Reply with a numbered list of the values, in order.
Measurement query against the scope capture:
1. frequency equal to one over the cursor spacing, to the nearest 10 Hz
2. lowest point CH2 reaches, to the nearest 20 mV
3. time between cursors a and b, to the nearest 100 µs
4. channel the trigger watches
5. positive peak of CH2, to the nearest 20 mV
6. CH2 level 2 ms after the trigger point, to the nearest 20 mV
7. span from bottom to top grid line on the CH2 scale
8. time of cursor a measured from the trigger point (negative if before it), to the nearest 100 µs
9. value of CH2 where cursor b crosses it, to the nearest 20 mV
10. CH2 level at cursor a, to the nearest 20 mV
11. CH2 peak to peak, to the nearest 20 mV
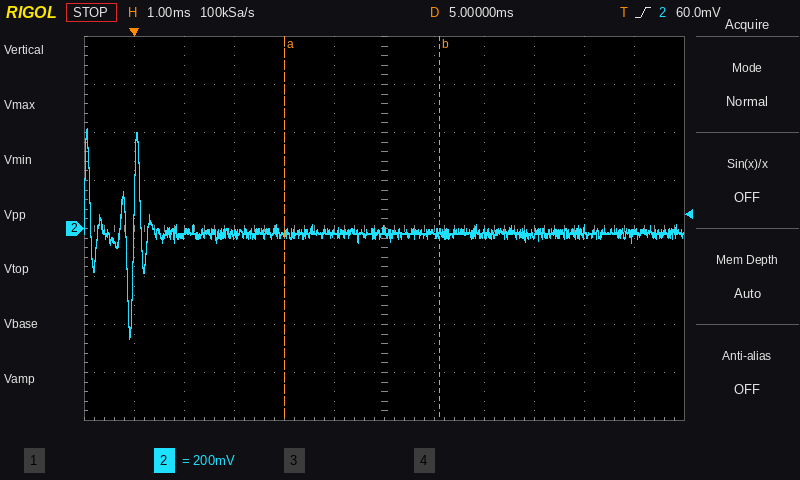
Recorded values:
1. 320 Hz
2. -460 mV
3. 3.1 ms
4. CH2
5. 420 mV
6. -20 mV
7. 1.6 V
8. +3.0 ms
9. -20 mV
10. -20 mV
11. 880 mV
